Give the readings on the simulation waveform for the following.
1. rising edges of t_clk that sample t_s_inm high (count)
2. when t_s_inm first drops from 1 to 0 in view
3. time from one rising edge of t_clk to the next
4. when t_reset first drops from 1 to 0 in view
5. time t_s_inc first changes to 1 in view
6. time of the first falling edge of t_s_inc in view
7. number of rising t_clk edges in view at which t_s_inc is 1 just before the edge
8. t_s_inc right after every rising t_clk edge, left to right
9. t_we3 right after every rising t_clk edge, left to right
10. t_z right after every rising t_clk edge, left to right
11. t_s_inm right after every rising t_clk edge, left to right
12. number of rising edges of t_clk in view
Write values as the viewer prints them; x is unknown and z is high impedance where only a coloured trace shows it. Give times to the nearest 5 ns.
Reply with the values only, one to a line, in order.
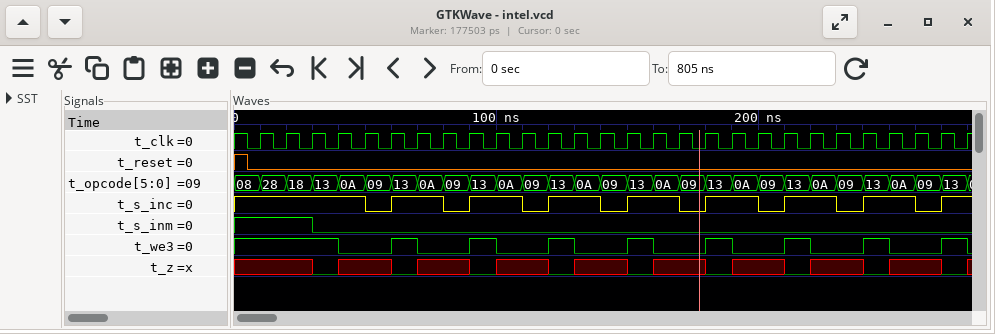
3
30 ns
10 ns
5 ns
60 ns
50 ns
20
1 1 1 1 0 1 1 0 1 1 0 1 1 0 1 1 0 1 1 0 1 1 0 1 1 0 1 1
1 1 1 0 0 1 0 0 1 0 0 1 0 0 1 0 0 1 0 0 1 0 0 1 0 0 1 0
x x 0 x x 0 x x 0 x x 0 x x 0 x x 0 x x 0 x x 0 x x 0 x
1 1 0 0 0 0 0 0 0 0 0 0 0 0 0 0 0 0 0 0 0 0 0 0 0 0 0 0
28
